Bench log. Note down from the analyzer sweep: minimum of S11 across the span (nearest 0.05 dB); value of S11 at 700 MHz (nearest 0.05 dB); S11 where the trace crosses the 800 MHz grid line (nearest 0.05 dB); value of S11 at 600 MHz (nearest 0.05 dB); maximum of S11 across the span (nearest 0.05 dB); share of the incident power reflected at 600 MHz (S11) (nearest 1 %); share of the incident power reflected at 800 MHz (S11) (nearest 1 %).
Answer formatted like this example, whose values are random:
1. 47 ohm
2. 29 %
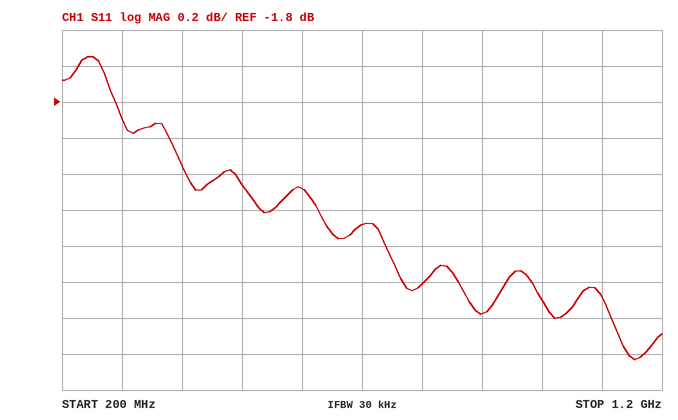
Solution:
1. -3.25 dB
2. -2.50 dB
3. -2.80 dB
4. -2.30 dB
5. -1.55 dB
6. 59 %
7. 52 %
